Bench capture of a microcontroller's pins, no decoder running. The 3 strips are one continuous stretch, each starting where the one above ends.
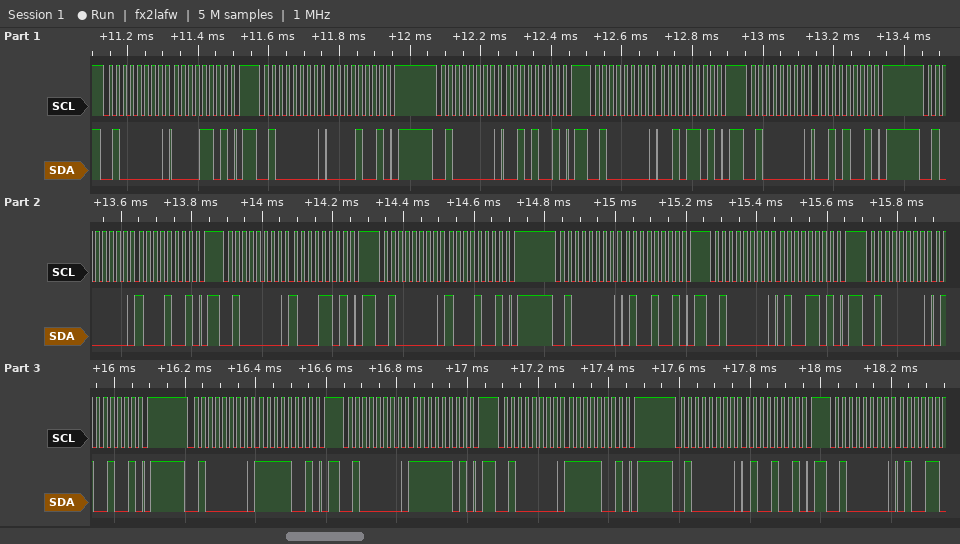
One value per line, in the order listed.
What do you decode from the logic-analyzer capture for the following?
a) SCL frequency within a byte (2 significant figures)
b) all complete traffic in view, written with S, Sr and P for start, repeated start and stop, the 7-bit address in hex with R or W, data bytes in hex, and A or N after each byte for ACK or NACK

50 kHz
S 20W A 0D A P S 20W A 09 A P S 20W A 29 A P S 20W A 2D A P S 20W A 29 A P S 20W A 89 A P S 20W A 8D A P S 20W A 89 A P S 20W A 49 A P S 20W A 4D A P S 20W A 49 A P S 20W A F9 A P S 20W A FD A P S 20W A F9 A P S 20W A 49 A P S 20W A
